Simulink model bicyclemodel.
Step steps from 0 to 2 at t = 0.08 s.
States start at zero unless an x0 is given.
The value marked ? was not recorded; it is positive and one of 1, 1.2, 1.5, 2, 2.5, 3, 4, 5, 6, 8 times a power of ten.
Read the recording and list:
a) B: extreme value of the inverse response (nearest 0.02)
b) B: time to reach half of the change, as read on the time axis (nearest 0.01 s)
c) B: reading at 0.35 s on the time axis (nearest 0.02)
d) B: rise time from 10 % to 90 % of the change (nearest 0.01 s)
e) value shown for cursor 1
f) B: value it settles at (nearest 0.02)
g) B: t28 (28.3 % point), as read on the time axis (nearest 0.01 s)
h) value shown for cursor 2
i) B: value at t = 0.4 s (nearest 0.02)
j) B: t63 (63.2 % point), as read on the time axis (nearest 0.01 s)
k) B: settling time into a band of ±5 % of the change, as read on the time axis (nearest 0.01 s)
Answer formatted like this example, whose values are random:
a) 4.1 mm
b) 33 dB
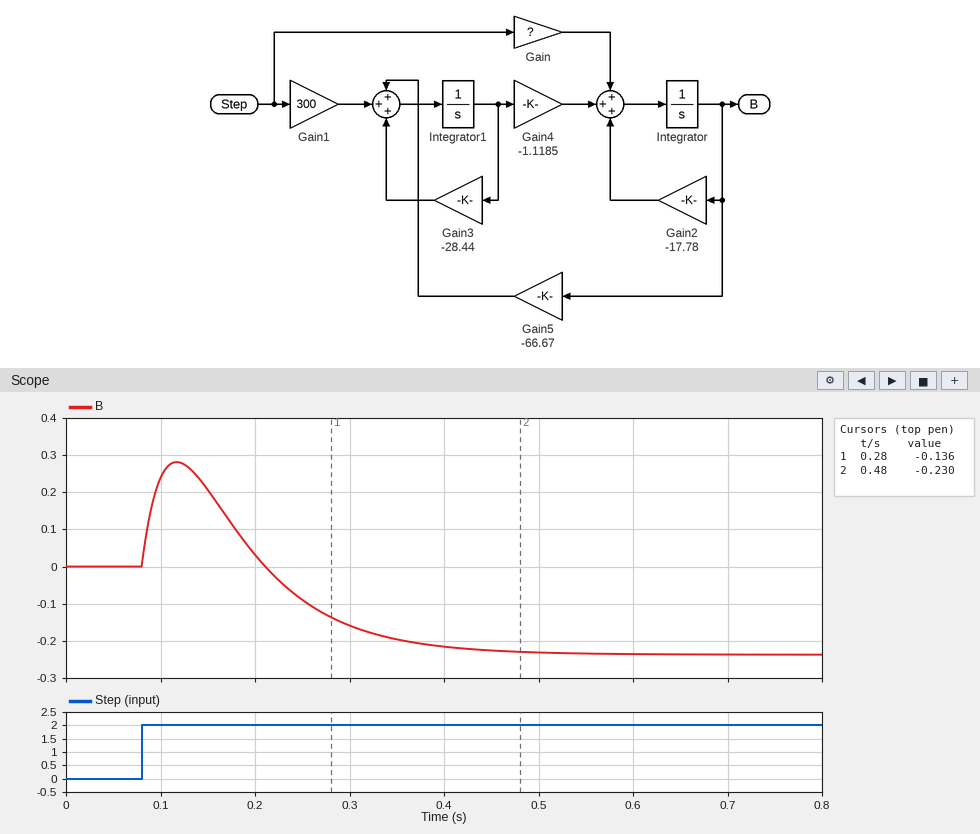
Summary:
a) 0.28
b) 0.27 s
c) -0.20
d) 0.17 s
e) -0.136
f) -0.24
g) 0.24 s
h) -0.230
i) -0.22
j) 0.29 s
k) 0.45 s
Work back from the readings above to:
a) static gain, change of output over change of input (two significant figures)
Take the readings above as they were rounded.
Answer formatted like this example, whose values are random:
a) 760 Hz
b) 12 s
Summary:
a) -0.12
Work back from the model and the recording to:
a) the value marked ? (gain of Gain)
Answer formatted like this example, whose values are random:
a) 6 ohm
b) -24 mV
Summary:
a) 10
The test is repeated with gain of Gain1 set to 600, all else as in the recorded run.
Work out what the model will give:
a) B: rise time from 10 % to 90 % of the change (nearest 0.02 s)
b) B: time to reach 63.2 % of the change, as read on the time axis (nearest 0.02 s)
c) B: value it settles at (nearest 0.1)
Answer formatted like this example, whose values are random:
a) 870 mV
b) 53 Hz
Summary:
a) 0.18 s
b) 0.22 s
c) -1.8
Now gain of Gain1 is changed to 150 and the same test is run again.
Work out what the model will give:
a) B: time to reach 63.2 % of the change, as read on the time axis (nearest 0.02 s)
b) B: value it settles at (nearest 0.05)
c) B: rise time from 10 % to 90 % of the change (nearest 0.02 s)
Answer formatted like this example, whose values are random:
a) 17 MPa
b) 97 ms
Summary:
a) 0.10 s
b) 0.55
c) 0.06 s
